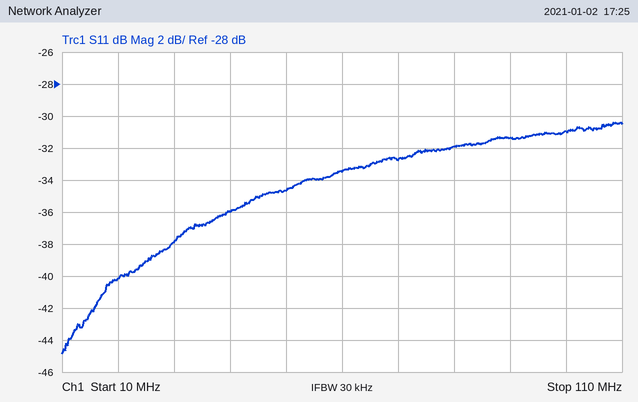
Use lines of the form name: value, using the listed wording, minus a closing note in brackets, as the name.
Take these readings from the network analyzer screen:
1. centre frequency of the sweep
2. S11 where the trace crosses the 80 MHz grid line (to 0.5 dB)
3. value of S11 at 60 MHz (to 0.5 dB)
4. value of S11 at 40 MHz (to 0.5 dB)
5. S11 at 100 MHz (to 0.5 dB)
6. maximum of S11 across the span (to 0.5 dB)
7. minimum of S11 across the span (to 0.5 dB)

centre frequency of the sweep: 60 MHz
S11 where the trace crosses the 80 MHz grid line: -32.0 dB
value of S11 at 60 MHz: -33.5 dB
value of S11 at 40 MHz: -36.0 dB
S11 at 100 MHz: -31.0 dB
maximum of S11 across the span: -30.5 dB
minimum of S11 across the span: -45.0 dB
